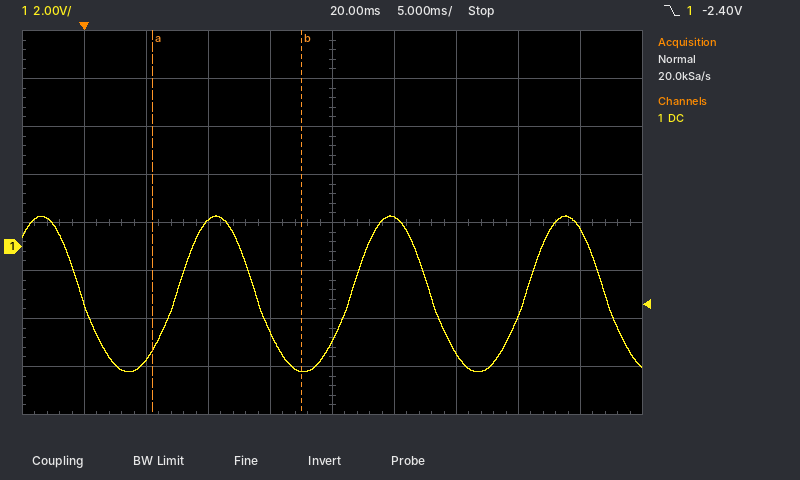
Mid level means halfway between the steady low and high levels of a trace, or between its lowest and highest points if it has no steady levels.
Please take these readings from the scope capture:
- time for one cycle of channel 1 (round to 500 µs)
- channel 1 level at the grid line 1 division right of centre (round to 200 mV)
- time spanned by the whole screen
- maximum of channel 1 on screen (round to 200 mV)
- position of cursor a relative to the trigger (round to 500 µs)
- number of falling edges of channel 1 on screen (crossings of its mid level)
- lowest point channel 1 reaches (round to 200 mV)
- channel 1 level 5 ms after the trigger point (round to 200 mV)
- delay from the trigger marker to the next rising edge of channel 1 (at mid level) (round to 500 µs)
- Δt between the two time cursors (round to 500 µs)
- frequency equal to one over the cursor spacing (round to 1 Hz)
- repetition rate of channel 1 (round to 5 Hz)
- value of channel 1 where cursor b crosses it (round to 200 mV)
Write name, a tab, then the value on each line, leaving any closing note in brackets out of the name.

time for one cycle of channel 1	14.0 ms
channel 1 level at the grid line 1 division right of centre	1.2 V
time spanned by the whole screen	50 ms
maximum of channel 1 on screen	1.2 V
position of cursor a relative to the trigger	+5.5 ms
number of falling edges of channel 1 on screen	4
lowest point channel 1 reaches	-5.2 V
channel 1 level 5 ms after the trigger point	-4.8 V
delay from the trigger marker to the next rising edge of channel 1 (at mid level)	7.5 ms
Δt between the two time cursors	12.0 ms
frequency equal to one over the cursor spacing	83 Hz
repetition rate of channel 1	70 Hz
value of channel 1 where cursor b crosses it	-5.2 V
